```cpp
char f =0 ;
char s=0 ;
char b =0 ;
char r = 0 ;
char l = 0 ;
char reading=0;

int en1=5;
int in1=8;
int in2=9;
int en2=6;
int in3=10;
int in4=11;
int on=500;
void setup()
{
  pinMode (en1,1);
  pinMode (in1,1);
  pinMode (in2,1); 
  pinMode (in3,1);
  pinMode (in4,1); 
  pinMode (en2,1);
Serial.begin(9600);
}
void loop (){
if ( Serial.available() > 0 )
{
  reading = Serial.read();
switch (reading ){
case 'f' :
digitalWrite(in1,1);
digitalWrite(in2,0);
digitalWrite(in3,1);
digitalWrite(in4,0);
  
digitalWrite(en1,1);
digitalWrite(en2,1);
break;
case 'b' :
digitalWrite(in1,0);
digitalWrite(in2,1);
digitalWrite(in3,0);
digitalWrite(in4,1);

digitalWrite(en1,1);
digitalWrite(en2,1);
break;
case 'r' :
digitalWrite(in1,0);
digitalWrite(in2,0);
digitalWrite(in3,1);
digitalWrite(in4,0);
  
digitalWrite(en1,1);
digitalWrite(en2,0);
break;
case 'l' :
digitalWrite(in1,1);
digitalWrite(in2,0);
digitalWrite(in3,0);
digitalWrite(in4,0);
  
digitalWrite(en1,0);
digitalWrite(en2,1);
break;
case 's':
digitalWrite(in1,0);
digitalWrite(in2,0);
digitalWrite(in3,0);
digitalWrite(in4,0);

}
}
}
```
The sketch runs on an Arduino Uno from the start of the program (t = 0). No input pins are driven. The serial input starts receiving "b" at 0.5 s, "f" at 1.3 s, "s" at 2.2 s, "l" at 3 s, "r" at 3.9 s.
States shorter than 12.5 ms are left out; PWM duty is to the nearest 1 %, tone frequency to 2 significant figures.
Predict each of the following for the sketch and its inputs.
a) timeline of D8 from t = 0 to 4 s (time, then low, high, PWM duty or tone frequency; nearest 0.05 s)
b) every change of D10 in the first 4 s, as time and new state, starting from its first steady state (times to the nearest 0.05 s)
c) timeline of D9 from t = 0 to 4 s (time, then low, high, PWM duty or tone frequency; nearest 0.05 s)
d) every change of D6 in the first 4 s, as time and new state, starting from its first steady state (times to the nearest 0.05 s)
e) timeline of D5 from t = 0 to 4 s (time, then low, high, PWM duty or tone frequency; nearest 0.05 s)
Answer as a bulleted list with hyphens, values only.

- 0 s low; 1.3 s high; 2.2 s low; 3 s high; 3.9 s low
- 0 s low; 1.3 s high; 2.2 s low; 3.9 s high
- 0 s low; 0.5 s high; 1.3 s low
- 0 s low; 0.5 s high; 3.9 s low
- 0 s low; 0.5 s high; 3 s low; 3.9 s high
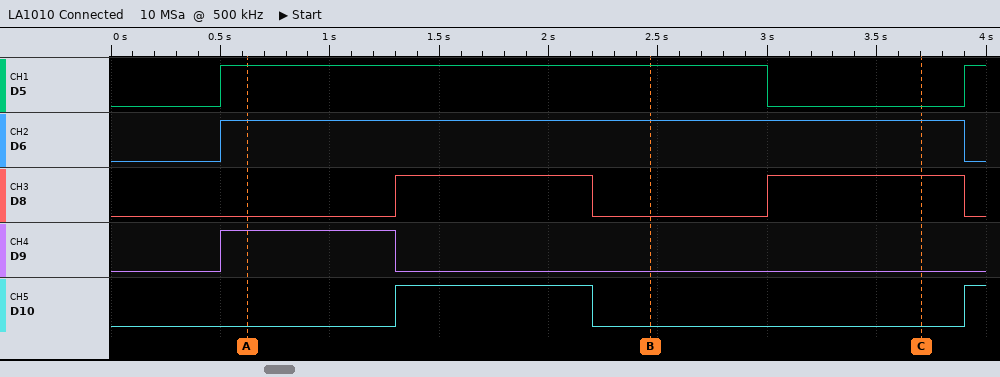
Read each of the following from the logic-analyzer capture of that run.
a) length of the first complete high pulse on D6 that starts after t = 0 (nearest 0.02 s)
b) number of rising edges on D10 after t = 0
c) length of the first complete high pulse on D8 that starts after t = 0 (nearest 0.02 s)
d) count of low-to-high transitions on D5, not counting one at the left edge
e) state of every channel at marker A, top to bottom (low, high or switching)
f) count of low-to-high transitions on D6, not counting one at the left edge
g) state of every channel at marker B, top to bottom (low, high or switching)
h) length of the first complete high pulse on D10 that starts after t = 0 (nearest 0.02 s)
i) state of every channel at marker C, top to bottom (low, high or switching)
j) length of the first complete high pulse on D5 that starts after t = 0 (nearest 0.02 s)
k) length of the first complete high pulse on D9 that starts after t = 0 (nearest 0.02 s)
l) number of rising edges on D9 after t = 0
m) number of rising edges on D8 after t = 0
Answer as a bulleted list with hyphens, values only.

- 3.40 s
- 2
- 0.90 s
- 2
- D5 high, D6 high, D8 low, D9 high, D10 low
- 1
- D5 high, D6 high, D8 low, D9 low, D10 low
- 0.90 s
- D5 low, D6 high, D8 high, D9 low, D10 low
- 2.50 s
- 0.80 s
- 1
- 2
